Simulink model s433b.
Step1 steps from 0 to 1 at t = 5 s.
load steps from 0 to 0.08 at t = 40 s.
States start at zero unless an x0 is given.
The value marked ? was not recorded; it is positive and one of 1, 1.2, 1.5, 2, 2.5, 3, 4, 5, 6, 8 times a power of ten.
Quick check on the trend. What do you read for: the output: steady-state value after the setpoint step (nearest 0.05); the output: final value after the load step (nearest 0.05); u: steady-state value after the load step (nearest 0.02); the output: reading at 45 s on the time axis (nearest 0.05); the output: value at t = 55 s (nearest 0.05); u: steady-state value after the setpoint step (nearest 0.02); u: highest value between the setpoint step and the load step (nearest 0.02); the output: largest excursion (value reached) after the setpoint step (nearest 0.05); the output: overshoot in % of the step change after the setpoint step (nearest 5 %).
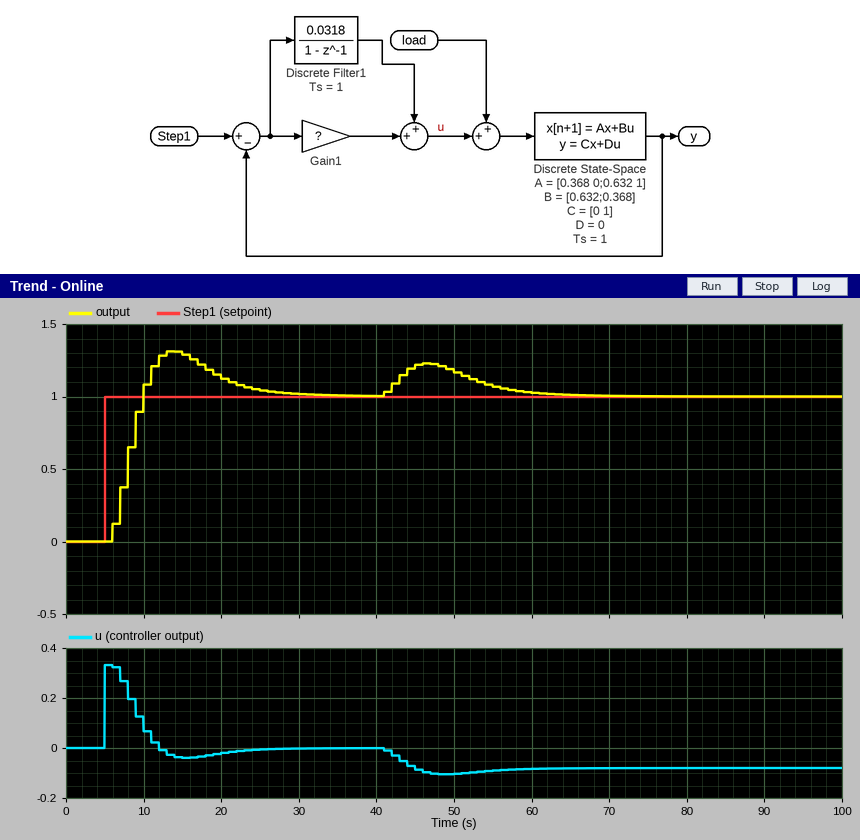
1.00
1.00
-0.08
1.20
1.05
0.00
0.34
1.30
30 %
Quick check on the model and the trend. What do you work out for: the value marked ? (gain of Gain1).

0.3
